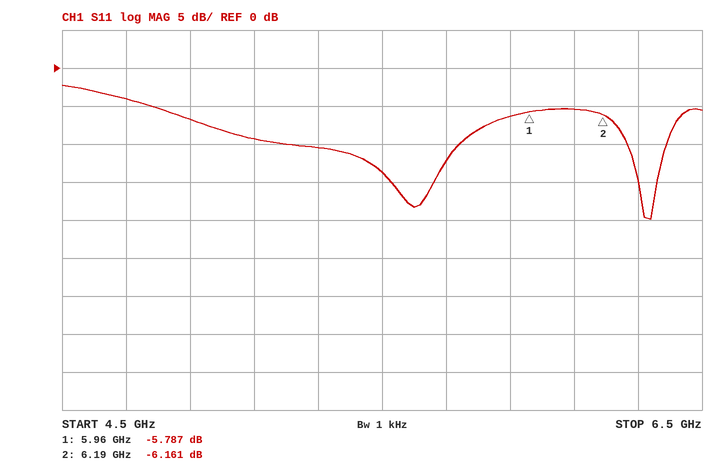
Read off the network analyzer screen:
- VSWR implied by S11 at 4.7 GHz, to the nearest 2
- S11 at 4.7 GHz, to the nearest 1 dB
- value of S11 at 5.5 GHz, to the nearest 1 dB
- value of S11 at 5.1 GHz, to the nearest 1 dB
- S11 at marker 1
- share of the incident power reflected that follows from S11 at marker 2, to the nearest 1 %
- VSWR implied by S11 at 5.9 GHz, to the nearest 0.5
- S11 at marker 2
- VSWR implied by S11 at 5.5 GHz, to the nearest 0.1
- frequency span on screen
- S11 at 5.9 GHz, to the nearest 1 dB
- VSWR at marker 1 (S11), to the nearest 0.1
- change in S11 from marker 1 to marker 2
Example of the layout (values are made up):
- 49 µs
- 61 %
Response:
- 4
- -4 dB
- -14 dB
- -9 dB
- -5.787 dB
- 24 %
- 3.0
- -6.161 dB
- 1.5
- 2 GHz
- -6 dB
- 3.1
- -0.374 dB
